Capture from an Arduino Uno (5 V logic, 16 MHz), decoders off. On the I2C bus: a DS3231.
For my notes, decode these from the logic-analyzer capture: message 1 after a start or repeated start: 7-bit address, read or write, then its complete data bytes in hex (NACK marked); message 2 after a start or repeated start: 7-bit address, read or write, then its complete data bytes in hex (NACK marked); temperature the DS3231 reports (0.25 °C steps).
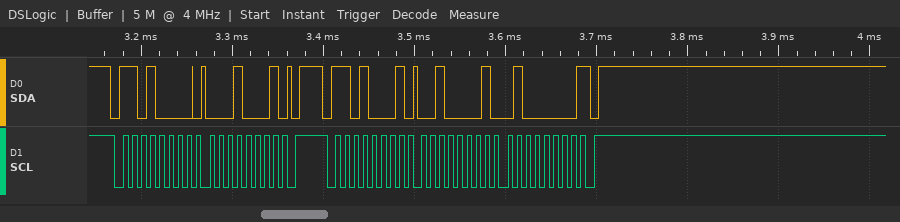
0x68 write: 11
0x68 read: 21 40 NACK
33.25 °C
